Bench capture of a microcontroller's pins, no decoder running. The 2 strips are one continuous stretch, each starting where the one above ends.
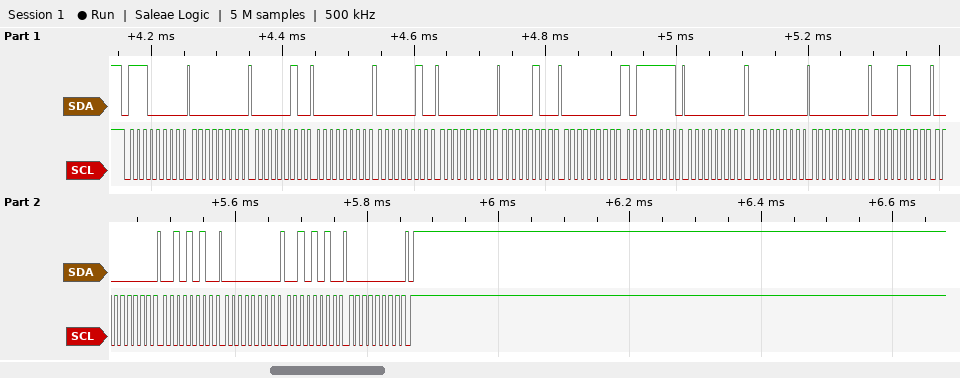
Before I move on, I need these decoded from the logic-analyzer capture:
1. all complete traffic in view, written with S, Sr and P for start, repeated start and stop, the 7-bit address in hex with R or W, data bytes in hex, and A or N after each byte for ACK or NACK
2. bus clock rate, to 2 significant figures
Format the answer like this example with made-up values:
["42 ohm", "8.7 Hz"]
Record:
["S 70W A 00 A 02 A 00 A 02 A 00 A 04 A 00 A BF A 00 A 00 A 00 A 0C A 00 A 2A A 00 A 2A A 00 A P", "100 kHz"]
